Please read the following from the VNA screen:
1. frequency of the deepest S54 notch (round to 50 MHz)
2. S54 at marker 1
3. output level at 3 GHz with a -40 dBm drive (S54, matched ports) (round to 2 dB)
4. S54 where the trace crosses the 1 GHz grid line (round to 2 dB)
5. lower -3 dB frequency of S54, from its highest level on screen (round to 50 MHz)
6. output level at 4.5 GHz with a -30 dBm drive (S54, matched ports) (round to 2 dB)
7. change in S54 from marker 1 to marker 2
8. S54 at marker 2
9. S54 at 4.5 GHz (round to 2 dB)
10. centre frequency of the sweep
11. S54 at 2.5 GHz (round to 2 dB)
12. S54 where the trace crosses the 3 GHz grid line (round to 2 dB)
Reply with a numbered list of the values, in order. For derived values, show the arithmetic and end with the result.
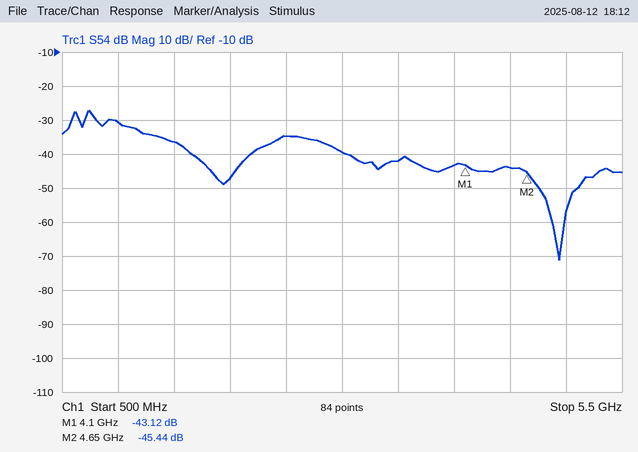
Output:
1. 4.95 GHz
2. -43.12 dB
3. -40 dBm + (-40 dB) = -80 dBm
4. -30 dB
5. 700 MHz
6. -30 dBm + (-44 dB) = -74 dBm
7. -45.44 − (-43.12) = -2.32 dB
8. -45.44 dB
9. -44 dB
10. 3 GHz
11. -34 dB
12. -40 dB
